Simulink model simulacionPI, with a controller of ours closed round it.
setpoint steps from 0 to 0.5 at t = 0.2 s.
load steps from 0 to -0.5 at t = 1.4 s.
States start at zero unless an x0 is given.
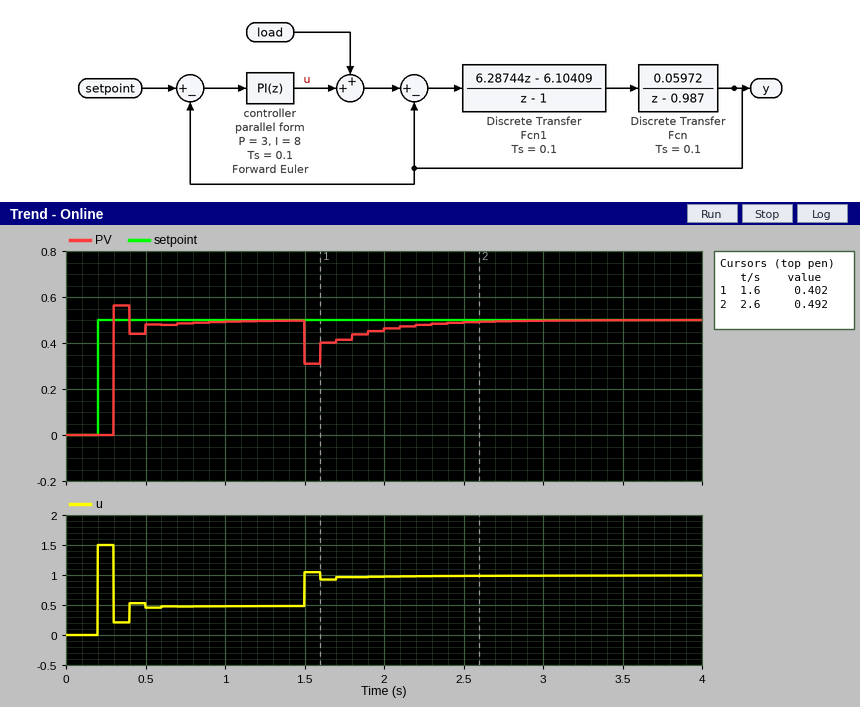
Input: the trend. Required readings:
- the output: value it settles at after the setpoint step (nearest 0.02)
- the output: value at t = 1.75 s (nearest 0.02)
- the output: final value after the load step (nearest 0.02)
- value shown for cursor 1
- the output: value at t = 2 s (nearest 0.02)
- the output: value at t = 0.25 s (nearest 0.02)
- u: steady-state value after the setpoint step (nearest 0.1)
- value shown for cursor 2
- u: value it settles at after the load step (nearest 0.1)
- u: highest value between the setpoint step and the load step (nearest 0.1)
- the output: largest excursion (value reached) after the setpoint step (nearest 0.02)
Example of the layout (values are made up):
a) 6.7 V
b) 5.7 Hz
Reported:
a) 0.50
b) 0.42
c) 0.50
d) 0.402
e) 0.46
f) 0.00
g) 0.5
h) 0.492
i) 1.0
j) 1.5
k) 0.56
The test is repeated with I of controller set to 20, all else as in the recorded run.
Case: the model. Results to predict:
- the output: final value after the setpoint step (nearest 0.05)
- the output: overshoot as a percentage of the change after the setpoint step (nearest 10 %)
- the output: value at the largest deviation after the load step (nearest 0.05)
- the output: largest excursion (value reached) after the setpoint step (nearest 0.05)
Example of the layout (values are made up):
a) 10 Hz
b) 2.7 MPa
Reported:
a) 0.50
b) 30 %
c) 0.30
d) 0.65
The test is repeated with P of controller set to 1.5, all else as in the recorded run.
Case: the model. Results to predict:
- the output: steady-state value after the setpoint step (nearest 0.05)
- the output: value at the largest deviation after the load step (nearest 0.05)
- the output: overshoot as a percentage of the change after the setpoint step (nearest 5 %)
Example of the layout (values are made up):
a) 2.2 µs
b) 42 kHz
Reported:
a) 0.50
b) 0.30
c) 10 %
